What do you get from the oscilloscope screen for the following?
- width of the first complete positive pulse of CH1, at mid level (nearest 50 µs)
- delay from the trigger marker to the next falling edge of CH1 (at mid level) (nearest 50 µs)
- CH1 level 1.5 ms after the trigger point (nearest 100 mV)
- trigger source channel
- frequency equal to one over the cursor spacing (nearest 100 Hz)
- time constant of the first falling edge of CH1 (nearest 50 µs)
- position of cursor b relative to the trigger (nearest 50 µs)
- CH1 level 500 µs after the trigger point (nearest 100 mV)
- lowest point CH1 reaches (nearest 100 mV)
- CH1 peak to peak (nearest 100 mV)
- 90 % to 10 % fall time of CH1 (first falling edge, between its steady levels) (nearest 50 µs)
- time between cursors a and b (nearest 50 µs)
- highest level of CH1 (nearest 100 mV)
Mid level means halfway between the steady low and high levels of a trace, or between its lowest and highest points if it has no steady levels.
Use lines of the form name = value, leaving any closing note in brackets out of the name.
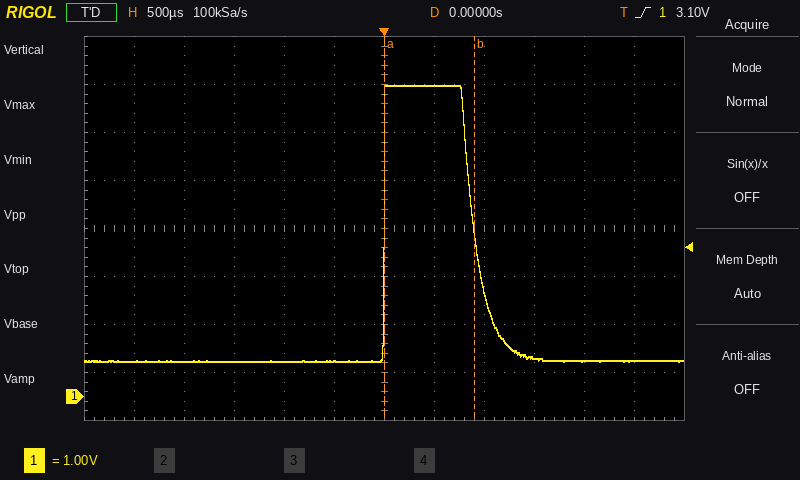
width of the first complete positive pulse of CH1, at mid level = 900 µs
delay from the trigger marker to the next falling edge of CH1 (at mid level) = 900 µs
CH1 level 1.5 ms after the trigger point = 800 mV
trigger source channel = CH1
frequency equal to one over the cursor spacing = 1.1 kHz
time constant of the first falling edge of CH1 = 150 µs
position of cursor b relative to the trigger = +900 µs
CH1 level 500 µs after the trigger point = 6.5 V
lowest point CH1 reaches = 700 mV
CH1 peak to peak = 5.8 V
90 % to 10 % fall time of CH1 (first falling edge, between its steady levels) = 350 µs
time between cursors a and b = 900 µs
highest level of CH1 = 6.5 V
